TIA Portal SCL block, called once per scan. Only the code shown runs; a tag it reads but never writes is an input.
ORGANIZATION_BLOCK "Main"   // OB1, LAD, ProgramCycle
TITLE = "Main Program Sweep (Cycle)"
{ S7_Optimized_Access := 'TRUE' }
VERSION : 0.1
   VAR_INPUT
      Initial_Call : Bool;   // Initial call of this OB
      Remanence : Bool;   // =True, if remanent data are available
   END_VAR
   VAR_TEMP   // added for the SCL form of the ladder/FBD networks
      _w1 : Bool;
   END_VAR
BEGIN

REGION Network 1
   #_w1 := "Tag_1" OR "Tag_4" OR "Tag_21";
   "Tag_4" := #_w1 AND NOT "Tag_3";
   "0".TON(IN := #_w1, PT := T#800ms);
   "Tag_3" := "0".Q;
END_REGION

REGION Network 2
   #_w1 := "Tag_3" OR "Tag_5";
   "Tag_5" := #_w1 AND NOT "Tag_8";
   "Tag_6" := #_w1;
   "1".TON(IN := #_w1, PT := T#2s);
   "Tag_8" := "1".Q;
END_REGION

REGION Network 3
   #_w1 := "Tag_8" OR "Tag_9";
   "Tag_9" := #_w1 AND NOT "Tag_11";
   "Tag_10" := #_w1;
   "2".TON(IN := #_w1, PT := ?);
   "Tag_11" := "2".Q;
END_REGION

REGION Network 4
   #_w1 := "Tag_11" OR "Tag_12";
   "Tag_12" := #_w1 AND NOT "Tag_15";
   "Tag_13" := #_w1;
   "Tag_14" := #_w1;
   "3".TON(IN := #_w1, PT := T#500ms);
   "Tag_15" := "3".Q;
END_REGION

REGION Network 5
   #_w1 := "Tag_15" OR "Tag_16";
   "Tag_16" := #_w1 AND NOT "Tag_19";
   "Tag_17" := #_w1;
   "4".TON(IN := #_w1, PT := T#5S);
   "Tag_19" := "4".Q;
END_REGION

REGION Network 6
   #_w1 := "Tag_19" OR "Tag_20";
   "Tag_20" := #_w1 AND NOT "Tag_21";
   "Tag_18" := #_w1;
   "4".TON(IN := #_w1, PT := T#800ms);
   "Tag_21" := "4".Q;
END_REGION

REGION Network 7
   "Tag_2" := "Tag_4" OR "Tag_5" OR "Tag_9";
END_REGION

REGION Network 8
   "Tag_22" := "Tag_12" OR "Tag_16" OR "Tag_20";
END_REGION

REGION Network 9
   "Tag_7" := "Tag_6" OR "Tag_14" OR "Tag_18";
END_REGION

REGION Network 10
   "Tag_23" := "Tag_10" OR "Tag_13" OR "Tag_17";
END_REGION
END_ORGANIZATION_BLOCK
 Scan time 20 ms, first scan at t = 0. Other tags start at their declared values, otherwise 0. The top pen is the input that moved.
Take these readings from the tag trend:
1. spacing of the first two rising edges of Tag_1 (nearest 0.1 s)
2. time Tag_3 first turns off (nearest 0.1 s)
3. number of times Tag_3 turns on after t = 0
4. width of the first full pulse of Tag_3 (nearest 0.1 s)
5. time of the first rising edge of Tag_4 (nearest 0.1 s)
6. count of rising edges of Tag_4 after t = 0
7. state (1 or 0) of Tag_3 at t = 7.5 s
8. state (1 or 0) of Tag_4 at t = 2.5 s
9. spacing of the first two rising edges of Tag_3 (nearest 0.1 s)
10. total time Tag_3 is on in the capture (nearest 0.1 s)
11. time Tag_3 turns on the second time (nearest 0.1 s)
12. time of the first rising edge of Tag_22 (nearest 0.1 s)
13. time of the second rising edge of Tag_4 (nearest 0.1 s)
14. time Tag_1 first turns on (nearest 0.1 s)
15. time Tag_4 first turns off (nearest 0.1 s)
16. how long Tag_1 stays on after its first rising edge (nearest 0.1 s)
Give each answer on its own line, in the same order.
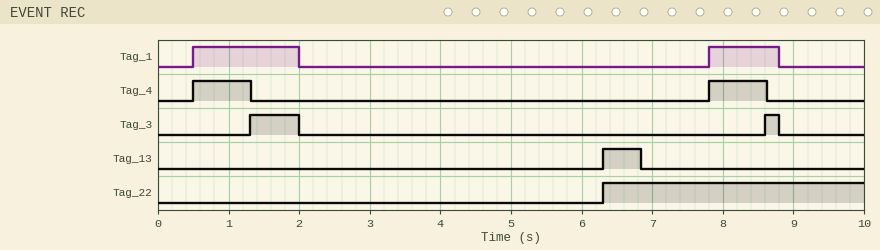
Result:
7.3 s
2.0 s
2
0.7 s
0.5 s
2
0
0
7.3 s
0.9 s
8.6 s
6.3 s
7.8 s
0.5 s
1.3 s
1.5 s
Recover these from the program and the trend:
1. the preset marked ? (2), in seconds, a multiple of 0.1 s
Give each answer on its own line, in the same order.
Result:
3.0 s
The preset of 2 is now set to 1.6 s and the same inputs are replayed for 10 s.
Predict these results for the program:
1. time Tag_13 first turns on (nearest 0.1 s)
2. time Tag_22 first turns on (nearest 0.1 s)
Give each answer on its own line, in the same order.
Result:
4.9 s
4.9 s
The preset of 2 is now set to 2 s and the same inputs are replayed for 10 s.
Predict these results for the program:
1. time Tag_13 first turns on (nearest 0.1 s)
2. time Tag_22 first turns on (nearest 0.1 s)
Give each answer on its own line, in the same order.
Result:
5.3 s
5.3 s
